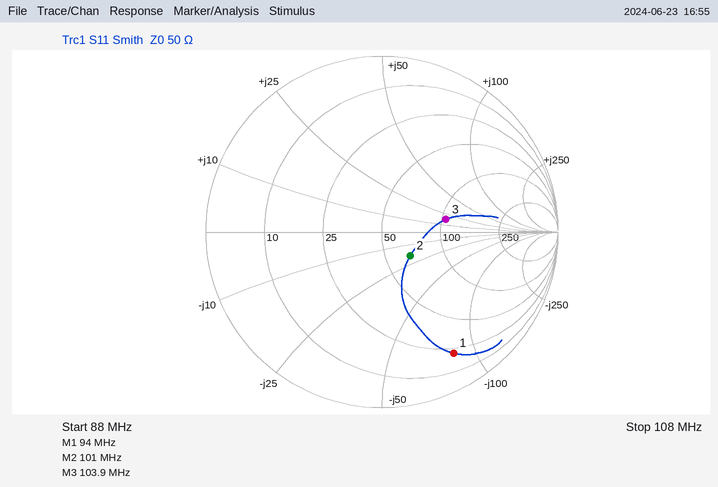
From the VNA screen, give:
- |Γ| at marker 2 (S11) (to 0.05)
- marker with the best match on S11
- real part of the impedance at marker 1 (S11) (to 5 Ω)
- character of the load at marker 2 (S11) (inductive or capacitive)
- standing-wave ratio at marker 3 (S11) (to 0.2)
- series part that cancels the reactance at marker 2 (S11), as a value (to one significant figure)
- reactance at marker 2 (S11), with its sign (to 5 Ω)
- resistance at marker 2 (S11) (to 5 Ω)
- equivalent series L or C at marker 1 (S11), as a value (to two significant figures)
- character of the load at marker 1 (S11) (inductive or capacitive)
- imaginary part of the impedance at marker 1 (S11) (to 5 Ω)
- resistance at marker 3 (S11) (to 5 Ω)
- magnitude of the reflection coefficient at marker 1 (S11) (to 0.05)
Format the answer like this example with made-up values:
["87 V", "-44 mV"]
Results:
["0.20", "marker 2", "20 Ω", "capacitive", "2.2", "30 nH", "-20 Ω", "65 Ω", "20 pF", "capacitive", "-85 Ω", "105 Ω", "0.80"]
